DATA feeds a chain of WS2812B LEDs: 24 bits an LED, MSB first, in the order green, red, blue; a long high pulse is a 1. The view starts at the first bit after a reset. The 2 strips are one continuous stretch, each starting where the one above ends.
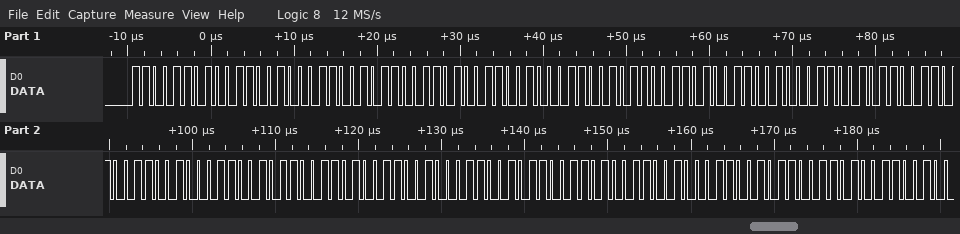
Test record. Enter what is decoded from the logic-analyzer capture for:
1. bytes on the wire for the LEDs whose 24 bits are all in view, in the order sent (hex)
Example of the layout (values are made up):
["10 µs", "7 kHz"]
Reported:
["CD 32 32 CD 32 32 CD 32 32 CD 32 32 CD 32 32 CD 32 32"]
